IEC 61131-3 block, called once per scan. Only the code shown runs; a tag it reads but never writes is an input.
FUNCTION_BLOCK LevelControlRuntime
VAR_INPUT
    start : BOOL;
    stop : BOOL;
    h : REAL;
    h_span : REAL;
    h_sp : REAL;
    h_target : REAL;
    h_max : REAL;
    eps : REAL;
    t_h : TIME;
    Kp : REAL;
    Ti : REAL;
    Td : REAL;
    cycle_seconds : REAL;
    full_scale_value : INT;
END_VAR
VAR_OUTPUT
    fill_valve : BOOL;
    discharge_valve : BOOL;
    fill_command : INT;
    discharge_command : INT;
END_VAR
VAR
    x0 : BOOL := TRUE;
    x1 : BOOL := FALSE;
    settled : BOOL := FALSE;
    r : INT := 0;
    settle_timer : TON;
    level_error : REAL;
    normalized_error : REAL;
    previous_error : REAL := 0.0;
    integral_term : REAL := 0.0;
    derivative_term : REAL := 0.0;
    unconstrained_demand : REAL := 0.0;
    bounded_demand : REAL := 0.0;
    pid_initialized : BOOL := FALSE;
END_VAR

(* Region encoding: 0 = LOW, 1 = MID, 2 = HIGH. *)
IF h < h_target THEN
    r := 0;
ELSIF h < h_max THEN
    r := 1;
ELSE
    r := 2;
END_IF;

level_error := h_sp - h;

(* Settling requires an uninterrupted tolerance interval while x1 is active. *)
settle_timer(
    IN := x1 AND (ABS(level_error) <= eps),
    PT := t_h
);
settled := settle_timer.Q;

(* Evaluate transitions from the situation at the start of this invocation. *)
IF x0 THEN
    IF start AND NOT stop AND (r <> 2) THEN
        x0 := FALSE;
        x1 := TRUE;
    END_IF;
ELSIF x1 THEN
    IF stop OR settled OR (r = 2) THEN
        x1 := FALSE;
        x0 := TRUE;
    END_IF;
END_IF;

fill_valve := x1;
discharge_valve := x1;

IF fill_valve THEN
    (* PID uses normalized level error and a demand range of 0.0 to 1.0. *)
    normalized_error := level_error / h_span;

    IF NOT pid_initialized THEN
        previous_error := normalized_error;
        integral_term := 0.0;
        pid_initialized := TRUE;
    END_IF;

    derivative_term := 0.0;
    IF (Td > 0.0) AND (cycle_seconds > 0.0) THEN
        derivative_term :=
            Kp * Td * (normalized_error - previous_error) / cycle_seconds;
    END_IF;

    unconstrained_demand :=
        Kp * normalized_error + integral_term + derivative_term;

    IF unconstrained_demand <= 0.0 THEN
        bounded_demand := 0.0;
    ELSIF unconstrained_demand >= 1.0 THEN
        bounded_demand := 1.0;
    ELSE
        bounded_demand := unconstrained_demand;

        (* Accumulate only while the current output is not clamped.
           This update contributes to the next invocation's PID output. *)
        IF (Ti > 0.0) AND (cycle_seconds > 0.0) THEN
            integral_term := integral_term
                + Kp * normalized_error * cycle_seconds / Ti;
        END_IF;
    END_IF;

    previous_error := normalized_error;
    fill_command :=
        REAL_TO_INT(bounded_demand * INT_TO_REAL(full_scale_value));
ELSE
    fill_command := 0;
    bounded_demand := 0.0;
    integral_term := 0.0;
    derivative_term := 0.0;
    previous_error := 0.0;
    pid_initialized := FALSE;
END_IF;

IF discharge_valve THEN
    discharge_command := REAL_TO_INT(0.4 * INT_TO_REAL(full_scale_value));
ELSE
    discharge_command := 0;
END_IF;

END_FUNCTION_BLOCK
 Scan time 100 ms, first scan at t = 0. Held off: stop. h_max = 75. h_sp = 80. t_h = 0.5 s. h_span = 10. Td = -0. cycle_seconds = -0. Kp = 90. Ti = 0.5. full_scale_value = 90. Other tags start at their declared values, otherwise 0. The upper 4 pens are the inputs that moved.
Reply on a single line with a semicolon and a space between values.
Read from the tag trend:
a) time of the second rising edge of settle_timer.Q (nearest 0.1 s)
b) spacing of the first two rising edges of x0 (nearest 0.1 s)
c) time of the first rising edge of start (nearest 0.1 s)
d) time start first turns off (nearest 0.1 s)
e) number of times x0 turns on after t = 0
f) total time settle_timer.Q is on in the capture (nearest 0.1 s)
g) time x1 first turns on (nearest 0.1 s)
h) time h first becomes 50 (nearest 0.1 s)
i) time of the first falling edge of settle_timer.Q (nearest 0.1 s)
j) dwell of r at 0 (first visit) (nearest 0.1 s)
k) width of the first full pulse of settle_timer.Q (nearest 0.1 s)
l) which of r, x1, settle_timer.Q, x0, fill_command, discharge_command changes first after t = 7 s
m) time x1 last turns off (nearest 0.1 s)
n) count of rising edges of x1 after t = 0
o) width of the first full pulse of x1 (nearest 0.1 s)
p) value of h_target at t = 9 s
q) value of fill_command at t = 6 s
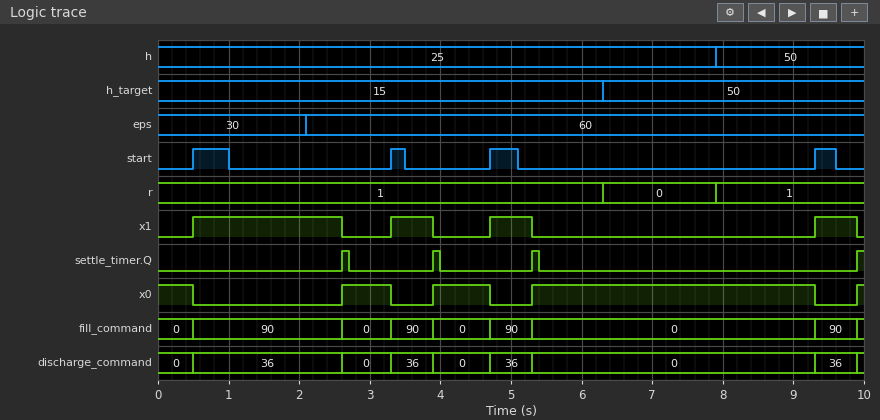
3.9 s; 1.3 s; 0.5 s; 1.0 s; 4; 0.4 s; 0.5 s; 7.9 s; 2.7 s; 1.6 s; 0.1 s; r; 9.9 s; 4; 2.1 s; 50; 0
